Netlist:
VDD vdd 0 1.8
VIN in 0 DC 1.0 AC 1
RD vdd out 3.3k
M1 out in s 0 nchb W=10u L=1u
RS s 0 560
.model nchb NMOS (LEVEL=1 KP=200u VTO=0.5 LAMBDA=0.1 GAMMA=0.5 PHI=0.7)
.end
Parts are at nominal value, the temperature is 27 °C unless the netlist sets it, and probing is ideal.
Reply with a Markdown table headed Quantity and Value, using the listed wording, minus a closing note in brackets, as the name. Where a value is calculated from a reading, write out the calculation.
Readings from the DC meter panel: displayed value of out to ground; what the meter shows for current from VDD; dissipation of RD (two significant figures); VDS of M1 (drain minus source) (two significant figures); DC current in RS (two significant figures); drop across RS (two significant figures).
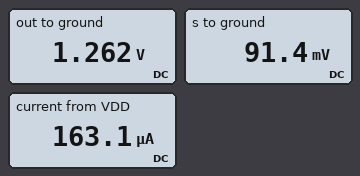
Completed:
| Quantity | Value |
|---|---|
| displayed value of out to ground | 1.262 V |
| what the meter shows for current from VDD | 163.1 µA |
| dissipation of RD | (1.8 V - 1.262 V)^2 / 3.3 kΩ = 88 µW |
| VDS of M1 (drain minus source) | 1.262 V - 91.4 mV = 1.2 V |
| DC current in RS | (91.4 mV) / 560 Ω = 160 µA |
| drop across RS | 91.4 mV = 91 mV |
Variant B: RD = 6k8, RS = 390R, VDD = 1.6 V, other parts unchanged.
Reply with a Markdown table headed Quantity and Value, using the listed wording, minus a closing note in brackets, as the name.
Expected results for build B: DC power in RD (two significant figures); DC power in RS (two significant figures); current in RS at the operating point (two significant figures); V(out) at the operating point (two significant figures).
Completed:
| Quantity | Value |
|---|---|
| DC power in RD | 200 µW |
| DC power in RS | 12 µW |
| current in RS at the operating point | 170 µA |
| V(out) at the operating point | 420 mV |
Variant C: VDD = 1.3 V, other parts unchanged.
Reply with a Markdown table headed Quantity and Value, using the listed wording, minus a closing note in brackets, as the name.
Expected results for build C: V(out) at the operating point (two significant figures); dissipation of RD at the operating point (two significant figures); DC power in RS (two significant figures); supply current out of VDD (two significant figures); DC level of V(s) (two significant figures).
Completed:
| Quantity | Value |
|---|---|
| V(out) at the operating point | 780 mV |
| dissipation of RD at the operating point | 83 µW |
| DC power in RS | 14 µW |
| supply current out of VDD | 160 µA |
| DC level of V(s) | 89 mV |
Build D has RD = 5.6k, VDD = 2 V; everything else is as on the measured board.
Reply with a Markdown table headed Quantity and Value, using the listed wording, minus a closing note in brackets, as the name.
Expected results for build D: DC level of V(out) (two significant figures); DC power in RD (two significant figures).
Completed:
| Quantity | Value |
|---|---|
| DC level of V(out) | 1.1 V |
| DC power in RD | 150 µW |
